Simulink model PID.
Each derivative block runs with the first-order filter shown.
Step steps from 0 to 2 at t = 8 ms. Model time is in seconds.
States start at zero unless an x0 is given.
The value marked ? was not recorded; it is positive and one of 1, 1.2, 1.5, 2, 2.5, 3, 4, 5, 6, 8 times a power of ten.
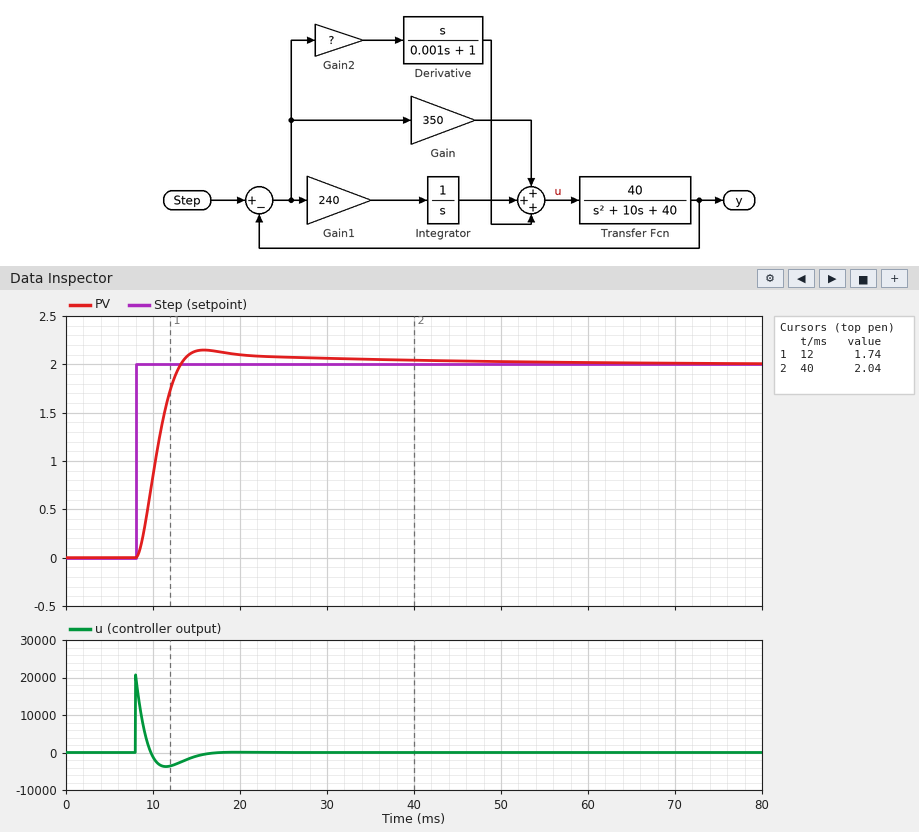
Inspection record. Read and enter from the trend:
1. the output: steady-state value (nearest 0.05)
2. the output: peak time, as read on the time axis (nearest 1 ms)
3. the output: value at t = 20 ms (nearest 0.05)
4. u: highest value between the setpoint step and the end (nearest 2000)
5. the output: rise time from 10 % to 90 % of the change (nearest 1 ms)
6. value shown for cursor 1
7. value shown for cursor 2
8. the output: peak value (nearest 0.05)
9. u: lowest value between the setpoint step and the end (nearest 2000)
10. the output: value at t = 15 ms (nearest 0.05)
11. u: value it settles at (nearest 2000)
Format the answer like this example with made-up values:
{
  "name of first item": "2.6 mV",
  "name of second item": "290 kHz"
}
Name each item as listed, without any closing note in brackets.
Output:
{
  "the output: steady-state value": "2.00",
  "the output: peak time, as read on the time axis": "16 ms",
  "the output: value at t = 20 ms": "2.10",
  "u: highest value between the setpoint step and the end": "20000",
  "the output: rise time from 10 % to 90 % of the change": "3 ms",
  "value shown for cursor 1": "1.74",
  "value shown for cursor 2": "2.04",
  "the output: peak value": "2.15",
  "u: lowest value between the setpoint step and the end": "-4000",
  "the output: value at t = 15 ms": "2.15",
  "u: value it settles at": "0"
}
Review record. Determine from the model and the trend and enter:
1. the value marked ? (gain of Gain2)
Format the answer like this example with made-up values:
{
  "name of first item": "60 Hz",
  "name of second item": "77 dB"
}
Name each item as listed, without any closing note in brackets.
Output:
{
  "the value marked ?": "10"
}
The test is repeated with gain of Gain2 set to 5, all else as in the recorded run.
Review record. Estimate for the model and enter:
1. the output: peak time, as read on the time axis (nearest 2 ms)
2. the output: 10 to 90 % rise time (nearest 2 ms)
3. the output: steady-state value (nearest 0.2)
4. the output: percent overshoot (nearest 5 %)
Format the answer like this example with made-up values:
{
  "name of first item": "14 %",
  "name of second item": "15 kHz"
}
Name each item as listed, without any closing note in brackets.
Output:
{
  "the output: peak time, as read on the time axis": "24 ms",
  "the output: 10 to 90 % rise time": "6 ms",
  "the output: steady-state value": "2.0",
  "the output: percent overshoot": "15 %"
}
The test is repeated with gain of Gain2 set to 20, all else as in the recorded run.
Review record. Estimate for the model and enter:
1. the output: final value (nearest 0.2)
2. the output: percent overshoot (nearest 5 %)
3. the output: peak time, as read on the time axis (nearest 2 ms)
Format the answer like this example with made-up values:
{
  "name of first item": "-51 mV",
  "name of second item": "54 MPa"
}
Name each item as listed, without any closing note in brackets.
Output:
{
  "the output: final value": "2.0",
  "the output: percent overshoot": "15 %",
  "the output: peak time, as read on the time axis": "12 ms"
}
